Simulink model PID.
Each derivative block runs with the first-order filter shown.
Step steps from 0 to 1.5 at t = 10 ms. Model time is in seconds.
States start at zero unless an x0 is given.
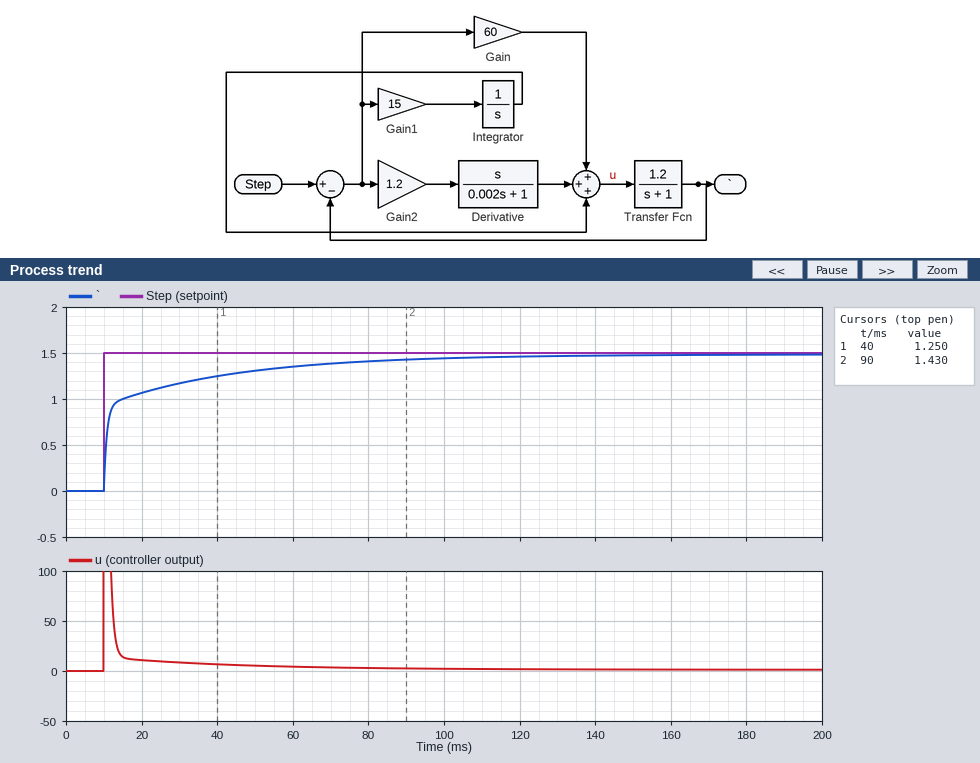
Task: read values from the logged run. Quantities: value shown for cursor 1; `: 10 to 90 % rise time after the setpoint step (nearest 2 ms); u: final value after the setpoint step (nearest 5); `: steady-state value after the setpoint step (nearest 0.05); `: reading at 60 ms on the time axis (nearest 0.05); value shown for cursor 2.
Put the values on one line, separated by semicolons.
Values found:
1.250; 46 ms; 0; 1.50; 1.35; 1.430
